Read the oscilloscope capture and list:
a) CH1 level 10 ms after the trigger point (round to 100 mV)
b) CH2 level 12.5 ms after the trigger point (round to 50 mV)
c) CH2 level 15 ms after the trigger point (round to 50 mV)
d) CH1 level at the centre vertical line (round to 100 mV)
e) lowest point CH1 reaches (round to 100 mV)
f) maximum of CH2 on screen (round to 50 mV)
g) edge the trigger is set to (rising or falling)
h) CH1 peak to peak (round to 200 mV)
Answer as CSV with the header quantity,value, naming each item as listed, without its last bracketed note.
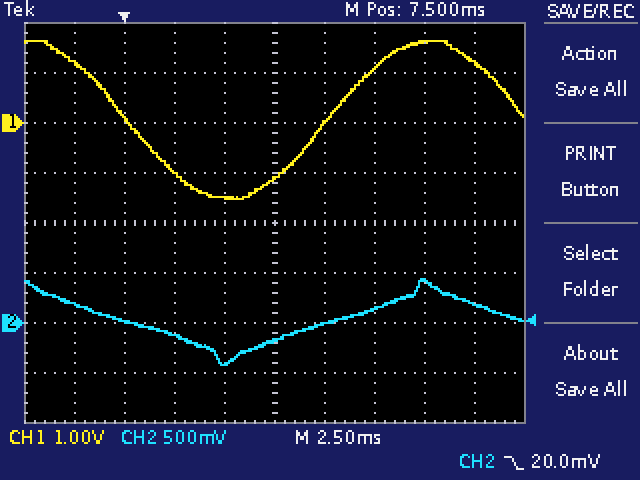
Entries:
quantity,value
CH1 level 10 ms after the trigger point,0.0 V
CH2 level 12.5 ms after the trigger point,150 mV
CH2 level 15 ms after the trigger point,400 mV
CH1 level at the centre vertical line,-1.1 V
lowest point CH1 reaches,-1.5 V
maximum of CH2 on screen,450 mV
edge the trigger is set to,falling
CH1 peak to peak,3.2 V
